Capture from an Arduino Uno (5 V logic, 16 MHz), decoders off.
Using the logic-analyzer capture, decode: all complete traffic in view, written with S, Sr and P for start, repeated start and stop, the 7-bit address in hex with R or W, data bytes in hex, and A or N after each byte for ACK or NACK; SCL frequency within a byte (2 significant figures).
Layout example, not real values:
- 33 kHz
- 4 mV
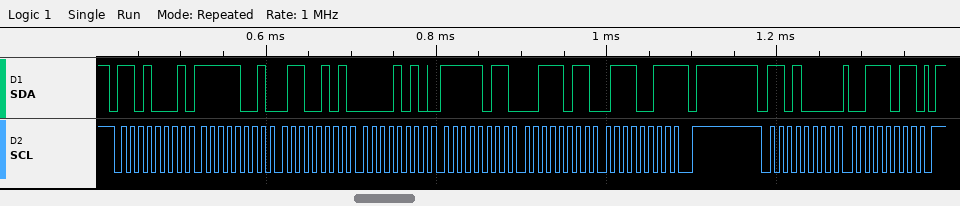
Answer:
- S 68R A F9 A 65 A 0A A FB A 3B A 73 N P S 68W A 3B A P
- 100 kHz
